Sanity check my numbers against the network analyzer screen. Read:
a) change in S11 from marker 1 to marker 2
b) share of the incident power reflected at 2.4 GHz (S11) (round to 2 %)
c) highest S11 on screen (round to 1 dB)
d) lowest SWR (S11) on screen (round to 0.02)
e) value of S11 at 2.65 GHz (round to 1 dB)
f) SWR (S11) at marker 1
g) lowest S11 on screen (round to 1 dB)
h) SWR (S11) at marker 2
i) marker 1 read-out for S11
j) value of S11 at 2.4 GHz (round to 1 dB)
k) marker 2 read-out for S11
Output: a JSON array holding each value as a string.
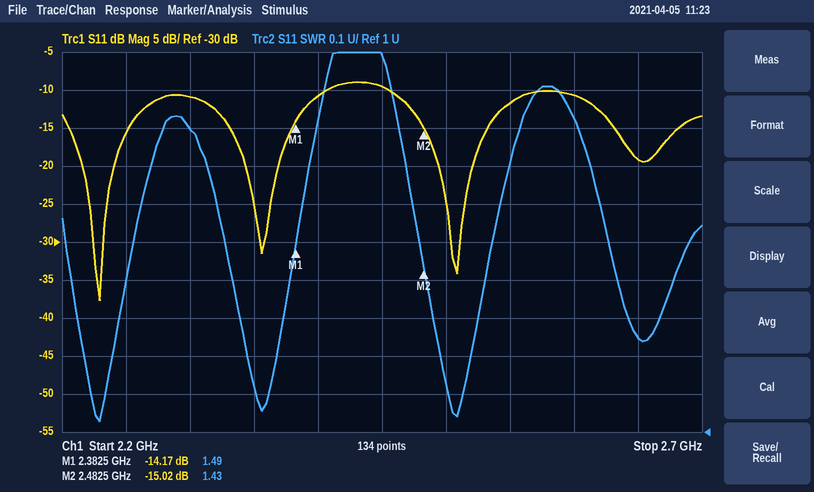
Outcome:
["-0.85 dB", "8 %", "-9 dB", "1.02", "-19 dB", "1.49", "-38 dB", "1.43", "-14.17 dB", "-11 dB", "-15.02 dB"]
